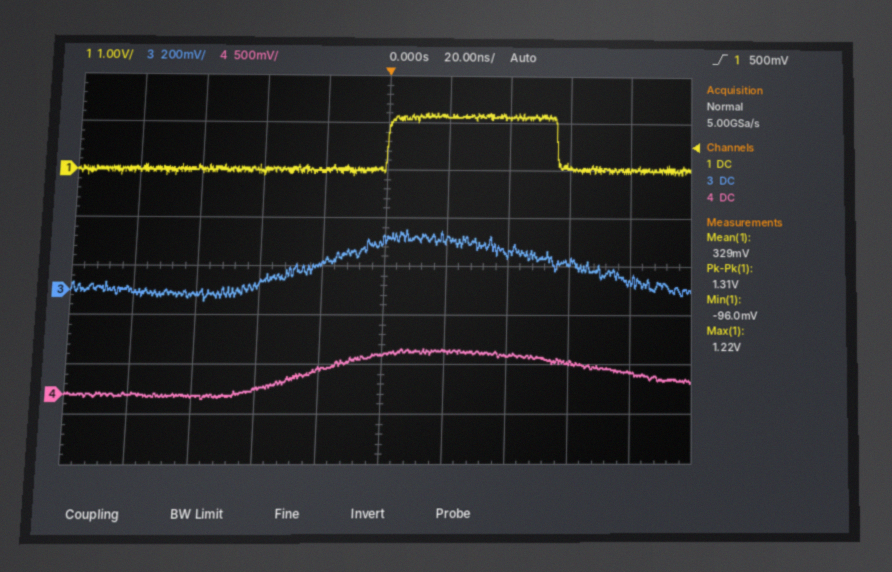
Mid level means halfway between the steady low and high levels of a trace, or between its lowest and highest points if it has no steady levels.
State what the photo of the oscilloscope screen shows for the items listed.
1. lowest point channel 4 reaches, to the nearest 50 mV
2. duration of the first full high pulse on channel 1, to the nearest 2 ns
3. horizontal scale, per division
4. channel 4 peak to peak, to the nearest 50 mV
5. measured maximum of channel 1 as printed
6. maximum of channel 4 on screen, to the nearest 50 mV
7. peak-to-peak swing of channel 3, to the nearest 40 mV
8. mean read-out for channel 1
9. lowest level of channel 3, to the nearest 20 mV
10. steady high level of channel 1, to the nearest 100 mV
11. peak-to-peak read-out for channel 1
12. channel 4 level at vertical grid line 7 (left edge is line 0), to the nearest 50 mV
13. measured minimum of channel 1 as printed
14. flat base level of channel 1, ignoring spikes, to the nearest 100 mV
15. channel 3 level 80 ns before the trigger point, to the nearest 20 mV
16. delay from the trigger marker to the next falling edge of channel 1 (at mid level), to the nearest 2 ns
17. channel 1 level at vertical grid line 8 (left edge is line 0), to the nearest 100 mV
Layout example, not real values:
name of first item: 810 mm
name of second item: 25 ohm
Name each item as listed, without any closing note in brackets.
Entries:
lowest point channel 4 reaches, to the nearest 50 mV: -50 mV
duration of the first full high pulse on channel 1, to the nearest 2 ns: 56 ns
horizontal scale, per division: 20 ns
channel 4 peak to peak, to the nearest 50 mV: 500 mV
measured maximum of channel 1 as printed: 1.22 V
maximum of channel 4 on screen, to the nearest 50 mV: 450 mV
peak-to-peak swing of channel 3, to the nearest 40 mV: 280 mV
mean read-out for channel 1: 329 mV
lowest level of channel 3, to the nearest 20 mV: -40 mV
steady high level of channel 1, to the nearest 100 mV: 1.1 V
peak-to-peak read-out for channel 1: 1.31 V
channel 4 level at vertical grid line 7 (left edge is line 0), to the nearest 50 mV: 400 mV
measured minimum of channel 1 as printed: -96.0 mV
flat base level of channel 1, ignoring spikes, to the nearest 100 mV: 0.0 V
channel 3 level 80 ns before the trigger point, to the nearest 20 mV: 0 mV
delay from the trigger marker to the next falling edge of channel 1 (at mid level), to the nearest 2 ns: 56 ns
channel 1 level at vertical grid line 8 (left edge is line 0), to the nearest 100 mV: 100 mV
